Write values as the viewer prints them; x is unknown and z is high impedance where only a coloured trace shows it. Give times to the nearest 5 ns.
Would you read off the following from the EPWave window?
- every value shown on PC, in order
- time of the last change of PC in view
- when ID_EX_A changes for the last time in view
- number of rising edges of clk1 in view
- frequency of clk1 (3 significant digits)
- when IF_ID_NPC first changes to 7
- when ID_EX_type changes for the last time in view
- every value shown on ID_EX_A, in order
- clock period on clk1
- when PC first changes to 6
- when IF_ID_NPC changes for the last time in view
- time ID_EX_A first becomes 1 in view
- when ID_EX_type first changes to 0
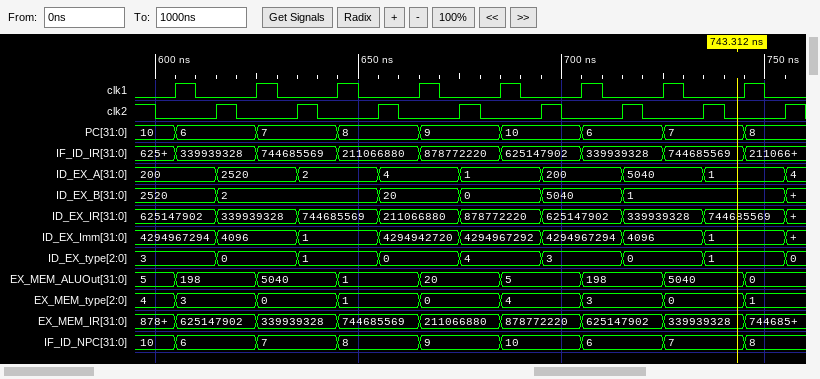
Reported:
10, 6, 7, 8, 9, 10, 6, 7, 8
745 ns
755 ns
8
50.0 MHz
625 ns
755 ns
200, 2520, 2, 4, 1, 200, 5040, 1, 4
20 ns
605 ns
745 ns
675 ns
615 ns
